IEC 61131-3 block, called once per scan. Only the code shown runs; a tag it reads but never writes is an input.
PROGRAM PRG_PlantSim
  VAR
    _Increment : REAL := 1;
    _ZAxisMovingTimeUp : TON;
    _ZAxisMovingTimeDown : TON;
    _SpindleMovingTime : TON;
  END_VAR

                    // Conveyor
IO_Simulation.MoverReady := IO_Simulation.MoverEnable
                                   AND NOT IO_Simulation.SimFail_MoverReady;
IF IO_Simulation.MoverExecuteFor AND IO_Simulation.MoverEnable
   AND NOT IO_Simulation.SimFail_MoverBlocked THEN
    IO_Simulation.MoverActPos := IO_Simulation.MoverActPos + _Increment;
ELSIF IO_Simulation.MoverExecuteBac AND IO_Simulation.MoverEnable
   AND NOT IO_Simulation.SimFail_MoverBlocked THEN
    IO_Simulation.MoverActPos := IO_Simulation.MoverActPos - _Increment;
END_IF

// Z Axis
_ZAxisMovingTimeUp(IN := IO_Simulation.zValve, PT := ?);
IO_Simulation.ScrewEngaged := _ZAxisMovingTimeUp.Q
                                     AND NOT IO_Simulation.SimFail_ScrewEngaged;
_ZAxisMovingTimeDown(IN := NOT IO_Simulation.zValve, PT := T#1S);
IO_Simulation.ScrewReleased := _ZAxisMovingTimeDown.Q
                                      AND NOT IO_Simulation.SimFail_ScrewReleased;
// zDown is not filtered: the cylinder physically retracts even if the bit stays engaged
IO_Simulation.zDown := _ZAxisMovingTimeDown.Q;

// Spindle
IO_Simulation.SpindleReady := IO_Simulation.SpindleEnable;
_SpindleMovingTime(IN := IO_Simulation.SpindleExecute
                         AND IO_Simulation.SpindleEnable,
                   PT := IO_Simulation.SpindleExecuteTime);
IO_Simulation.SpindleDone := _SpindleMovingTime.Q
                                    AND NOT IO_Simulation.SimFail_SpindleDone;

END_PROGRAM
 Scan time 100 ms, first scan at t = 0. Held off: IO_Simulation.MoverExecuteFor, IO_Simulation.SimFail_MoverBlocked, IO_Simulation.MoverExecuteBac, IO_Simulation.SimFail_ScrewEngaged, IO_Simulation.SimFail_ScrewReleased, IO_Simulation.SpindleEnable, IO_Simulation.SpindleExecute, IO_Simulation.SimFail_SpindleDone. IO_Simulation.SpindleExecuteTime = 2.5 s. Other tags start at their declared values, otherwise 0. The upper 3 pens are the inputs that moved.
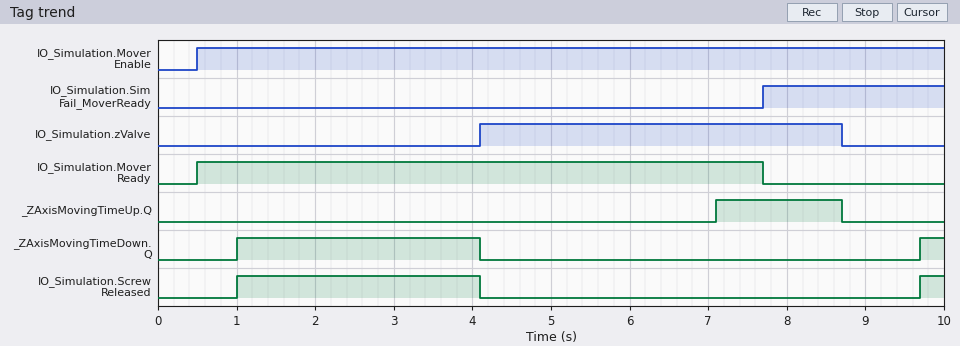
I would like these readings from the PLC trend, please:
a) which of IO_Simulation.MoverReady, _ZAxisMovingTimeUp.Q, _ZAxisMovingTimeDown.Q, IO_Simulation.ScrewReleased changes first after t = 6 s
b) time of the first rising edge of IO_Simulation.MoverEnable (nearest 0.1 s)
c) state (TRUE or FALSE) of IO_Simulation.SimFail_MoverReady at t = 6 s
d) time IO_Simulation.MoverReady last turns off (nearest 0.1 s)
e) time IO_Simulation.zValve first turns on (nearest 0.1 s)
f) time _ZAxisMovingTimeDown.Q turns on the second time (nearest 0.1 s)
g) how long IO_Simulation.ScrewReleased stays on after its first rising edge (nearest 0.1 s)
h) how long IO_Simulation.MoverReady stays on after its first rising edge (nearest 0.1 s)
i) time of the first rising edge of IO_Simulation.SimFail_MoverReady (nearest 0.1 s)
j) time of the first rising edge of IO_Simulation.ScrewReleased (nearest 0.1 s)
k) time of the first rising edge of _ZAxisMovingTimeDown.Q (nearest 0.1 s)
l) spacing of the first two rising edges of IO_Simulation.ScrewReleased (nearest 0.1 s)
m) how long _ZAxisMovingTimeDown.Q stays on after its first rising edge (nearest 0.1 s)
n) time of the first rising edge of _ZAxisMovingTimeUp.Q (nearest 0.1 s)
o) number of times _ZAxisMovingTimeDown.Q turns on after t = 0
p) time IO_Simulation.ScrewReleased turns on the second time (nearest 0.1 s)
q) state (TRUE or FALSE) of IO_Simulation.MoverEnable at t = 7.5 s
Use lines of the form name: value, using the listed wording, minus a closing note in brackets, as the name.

which of IO_Simulation.MoverReady, _ZAxisMovingTimeUp.Q, _ZAxisMovingTimeDown.Q, IO_Simulation.ScrewReleased changes first after t = 6 s: _ZAxisMovingTimeUp.Q
time of the first rising edge of IO_Simulation.MoverEnable: 0.5 s
state (TRUE or FALSE) of IO_Simulation.SimFail_MoverReady at t = 6 s: FALSE
time IO_Simulation.MoverReady last turns off: 7.7 s
time IO_Simulation.zValve first turns on: 4.1 s
time _ZAxisMovingTimeDown.Q turns on the second time: 9.7 s
how long IO_Simulation.ScrewReleased stays on after its first rising edge: 3.1 s
how long IO_Simulation.MoverReady stays on after its first rising edge: 7.2 s
time of the first rising edge of IO_Simulation.SimFail_MoverReady: 7.7 s
time of the first rising edge of IO_Simulation.ScrewReleased: 1.0 s
time of the first rising edge of _ZAxisMovingTimeDown.Q: 1.0 s
spacing of the first two rising edges of IO_Simulation.ScrewReleased: 8.7 s
how long _ZAxisMovingTimeDown.Q stays on after its first rising edge: 3.1 s
time of the first rising edge of _ZAxisMovingTimeUp.Q: 7.1 s
number of times _ZAxisMovingTimeDown.Q turns on after t = 0: 2
time IO_Simulation.ScrewReleased turns on the second time: 9.7 s
state (TRUE or FALSE) of IO_Simulation.MoverEnable at t = 7.5 s: TRUE
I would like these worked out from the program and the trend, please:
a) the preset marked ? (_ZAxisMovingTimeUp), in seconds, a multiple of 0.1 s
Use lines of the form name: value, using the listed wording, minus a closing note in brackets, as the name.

the preset marked ? (_ZAxisMovingTimeUp), in seconds, a multiple of 0.1 s: 3.0 s
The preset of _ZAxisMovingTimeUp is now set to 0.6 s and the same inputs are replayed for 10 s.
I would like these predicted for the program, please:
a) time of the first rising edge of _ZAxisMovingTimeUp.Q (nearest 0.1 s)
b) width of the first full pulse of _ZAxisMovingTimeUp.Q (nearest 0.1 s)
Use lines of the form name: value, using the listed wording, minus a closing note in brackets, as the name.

time of the first rising edge of _ZAxisMovingTimeUp.Q: 4.7 s
width of the first full pulse of _ZAxisMovingTimeUp.Q: 4.0 s
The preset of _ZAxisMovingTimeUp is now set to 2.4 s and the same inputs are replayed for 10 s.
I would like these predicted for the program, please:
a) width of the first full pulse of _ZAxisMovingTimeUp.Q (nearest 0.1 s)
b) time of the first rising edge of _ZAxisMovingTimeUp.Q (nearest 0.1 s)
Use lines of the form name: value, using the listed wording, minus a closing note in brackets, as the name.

width of the first full pulse of _ZAxisMovingTimeUp.Q: 2.2 s
time of the first rising edge of _ZAxisMovingTimeUp.Q: 6.5 s
